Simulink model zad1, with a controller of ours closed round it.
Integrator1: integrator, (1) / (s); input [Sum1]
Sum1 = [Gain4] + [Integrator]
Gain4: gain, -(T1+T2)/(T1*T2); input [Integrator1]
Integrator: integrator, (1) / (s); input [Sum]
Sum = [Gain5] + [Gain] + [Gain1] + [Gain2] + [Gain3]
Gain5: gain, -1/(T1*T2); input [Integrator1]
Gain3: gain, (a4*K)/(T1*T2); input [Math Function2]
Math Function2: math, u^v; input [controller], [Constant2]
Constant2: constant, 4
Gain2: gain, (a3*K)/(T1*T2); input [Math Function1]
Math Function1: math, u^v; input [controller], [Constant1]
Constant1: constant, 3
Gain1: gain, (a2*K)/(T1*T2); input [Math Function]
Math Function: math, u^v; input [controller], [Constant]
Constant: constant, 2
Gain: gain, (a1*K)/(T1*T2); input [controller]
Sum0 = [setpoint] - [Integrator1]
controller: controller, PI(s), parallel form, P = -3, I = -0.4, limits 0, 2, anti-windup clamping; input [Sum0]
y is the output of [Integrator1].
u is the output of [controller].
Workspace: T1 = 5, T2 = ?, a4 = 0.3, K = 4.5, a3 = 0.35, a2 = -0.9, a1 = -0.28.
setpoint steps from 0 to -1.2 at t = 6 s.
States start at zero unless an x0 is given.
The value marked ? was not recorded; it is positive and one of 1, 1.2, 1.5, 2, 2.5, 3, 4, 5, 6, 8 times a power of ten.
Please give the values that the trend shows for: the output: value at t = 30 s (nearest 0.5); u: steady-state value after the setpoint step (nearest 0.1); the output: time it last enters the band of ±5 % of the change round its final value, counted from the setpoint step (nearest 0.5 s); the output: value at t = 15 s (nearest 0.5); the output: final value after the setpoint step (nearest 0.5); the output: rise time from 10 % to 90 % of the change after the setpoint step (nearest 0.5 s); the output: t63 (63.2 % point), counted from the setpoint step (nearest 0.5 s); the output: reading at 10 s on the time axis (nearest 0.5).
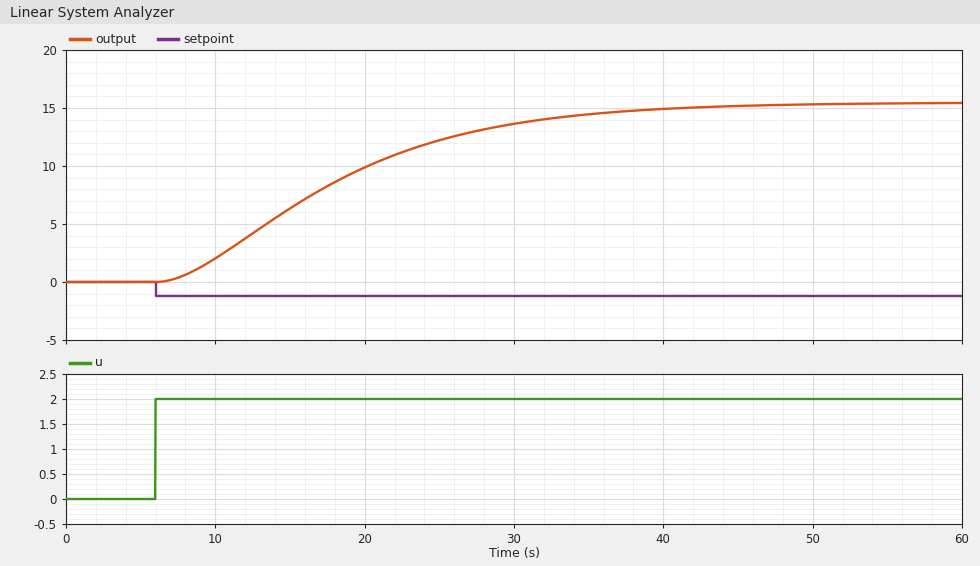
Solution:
13.5
2.0
31.5 s
6.5
15.5
22.0 s
14.0 s
2.0
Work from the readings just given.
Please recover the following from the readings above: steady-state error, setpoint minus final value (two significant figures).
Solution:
-17
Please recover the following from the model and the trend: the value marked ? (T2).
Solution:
8
